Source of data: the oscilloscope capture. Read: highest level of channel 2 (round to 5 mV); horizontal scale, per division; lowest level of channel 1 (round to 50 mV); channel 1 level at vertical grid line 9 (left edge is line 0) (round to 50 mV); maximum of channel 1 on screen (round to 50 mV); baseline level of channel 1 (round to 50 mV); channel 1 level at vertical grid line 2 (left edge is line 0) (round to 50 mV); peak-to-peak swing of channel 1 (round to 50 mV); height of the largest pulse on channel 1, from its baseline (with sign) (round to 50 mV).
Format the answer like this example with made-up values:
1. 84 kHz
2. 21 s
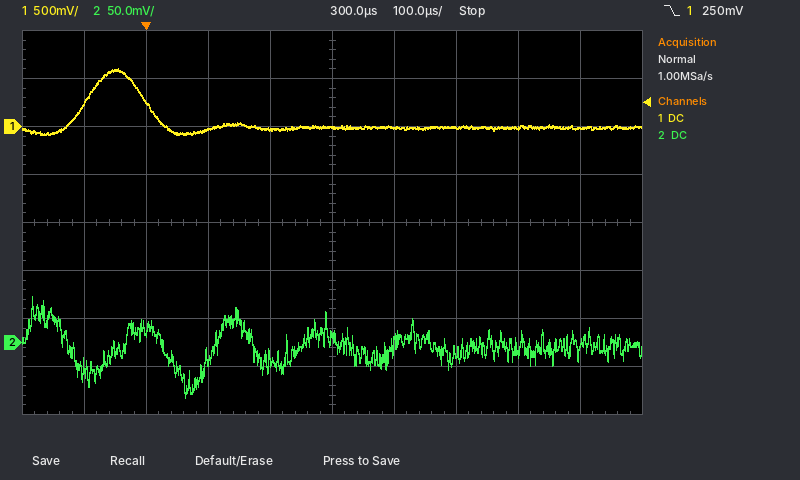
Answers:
1. 50 mV
2. 100 µs
3. -100 mV
4. 0 mV
5. 600 mV
6. 0 mV
7. 250 mV
8. 700 mV
9. +600 mV
